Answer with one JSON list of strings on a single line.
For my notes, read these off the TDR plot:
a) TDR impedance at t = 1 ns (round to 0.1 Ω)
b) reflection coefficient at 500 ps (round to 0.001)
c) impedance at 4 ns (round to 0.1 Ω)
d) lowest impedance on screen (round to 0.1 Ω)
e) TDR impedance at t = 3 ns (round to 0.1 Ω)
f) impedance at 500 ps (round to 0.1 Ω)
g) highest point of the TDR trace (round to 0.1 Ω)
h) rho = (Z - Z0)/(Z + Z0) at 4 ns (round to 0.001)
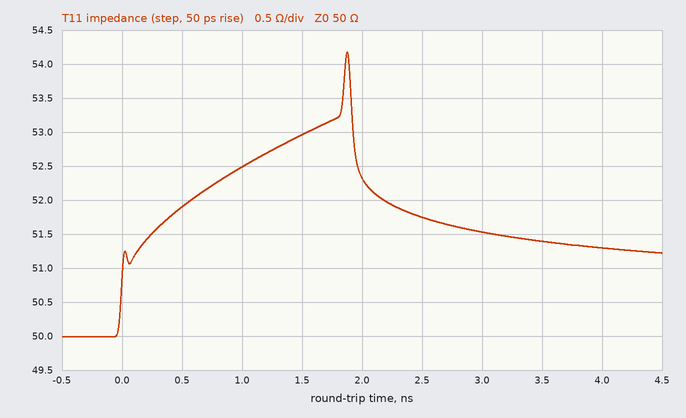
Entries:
["52.5 Ω", "+0.019", "51.3 Ω", "50.0 Ω", "51.5 Ω", "51.9 Ω", "54.2 Ω", "+0.013"]
